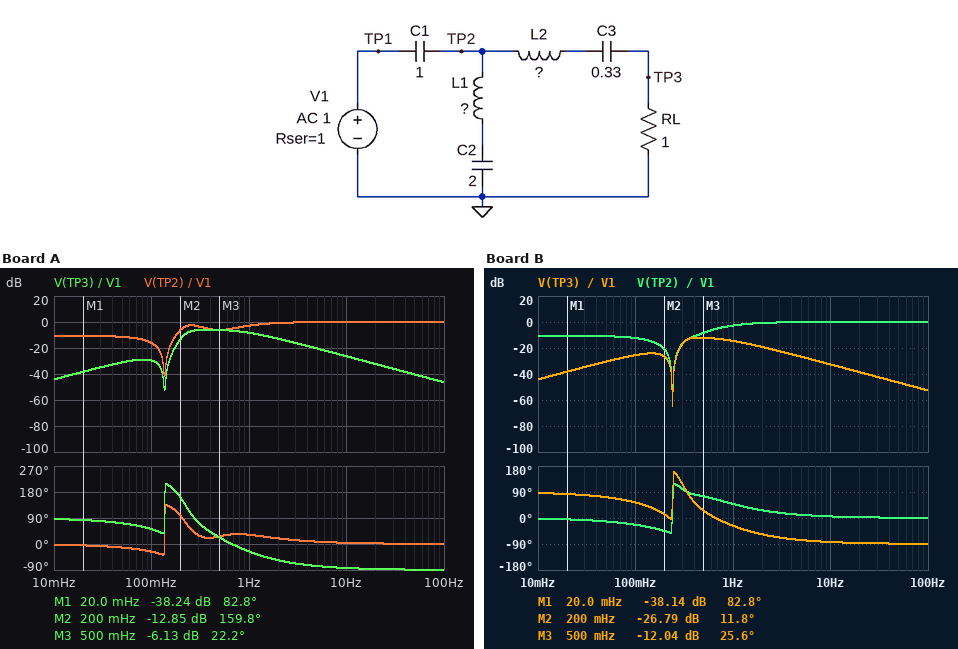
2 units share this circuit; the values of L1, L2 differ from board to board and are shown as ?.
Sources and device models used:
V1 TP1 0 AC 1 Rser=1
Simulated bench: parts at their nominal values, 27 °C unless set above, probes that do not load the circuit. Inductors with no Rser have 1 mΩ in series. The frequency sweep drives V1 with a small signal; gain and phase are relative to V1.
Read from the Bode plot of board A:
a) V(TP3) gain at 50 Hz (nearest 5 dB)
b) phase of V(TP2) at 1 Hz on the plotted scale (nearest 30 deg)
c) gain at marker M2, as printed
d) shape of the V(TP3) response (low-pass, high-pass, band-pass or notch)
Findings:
-40 dB
30 deg
-12.85 dB
band-pass
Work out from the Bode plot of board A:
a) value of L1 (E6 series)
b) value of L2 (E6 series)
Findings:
680 mH
330 mH
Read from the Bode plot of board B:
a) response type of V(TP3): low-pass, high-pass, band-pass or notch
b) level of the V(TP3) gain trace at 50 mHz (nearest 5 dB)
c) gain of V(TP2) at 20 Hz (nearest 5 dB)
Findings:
band-pass
-30 dB
0 dB
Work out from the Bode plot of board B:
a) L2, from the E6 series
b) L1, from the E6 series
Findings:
680 mH
220 mH
